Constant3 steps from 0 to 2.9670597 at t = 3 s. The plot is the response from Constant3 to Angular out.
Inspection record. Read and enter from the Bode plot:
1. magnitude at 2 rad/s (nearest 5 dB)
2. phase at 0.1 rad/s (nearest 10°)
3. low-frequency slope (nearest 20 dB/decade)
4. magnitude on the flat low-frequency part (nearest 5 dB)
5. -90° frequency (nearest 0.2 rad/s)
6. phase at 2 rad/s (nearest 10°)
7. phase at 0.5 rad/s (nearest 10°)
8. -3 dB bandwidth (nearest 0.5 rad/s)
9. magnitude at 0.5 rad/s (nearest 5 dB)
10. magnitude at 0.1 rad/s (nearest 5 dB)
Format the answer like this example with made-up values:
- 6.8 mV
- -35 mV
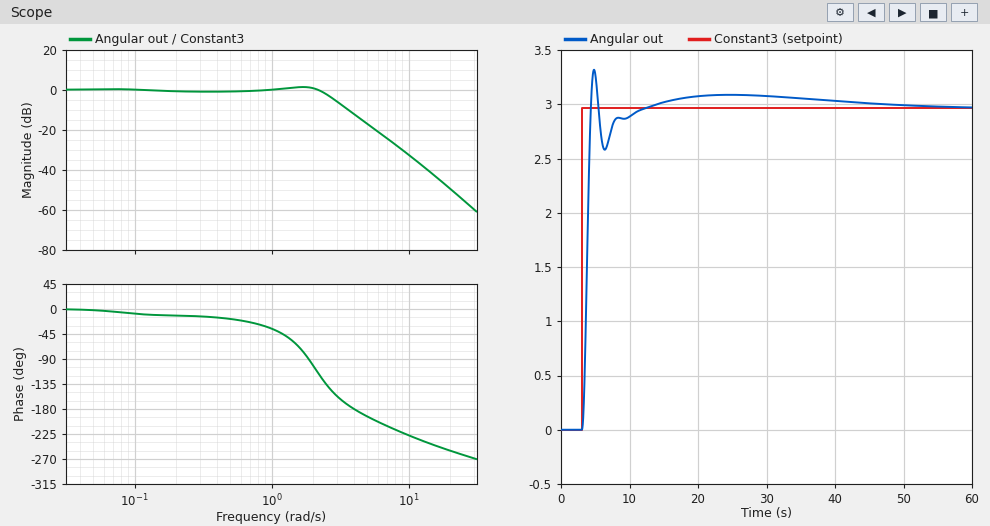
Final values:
- 0 dB
- -10°
- 0 dB/decade
- 0 dB
- 1.8 rad/s
- -100°
- -20°
- 2.5 rad/s
- 0 dB
- 0 dB
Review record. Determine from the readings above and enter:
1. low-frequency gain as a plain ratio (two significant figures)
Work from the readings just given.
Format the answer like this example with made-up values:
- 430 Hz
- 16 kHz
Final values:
- 1.0
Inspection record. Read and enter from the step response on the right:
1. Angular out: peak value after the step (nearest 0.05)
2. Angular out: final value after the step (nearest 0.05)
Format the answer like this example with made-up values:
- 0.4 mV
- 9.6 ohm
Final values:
- 3.30
- 2.95
